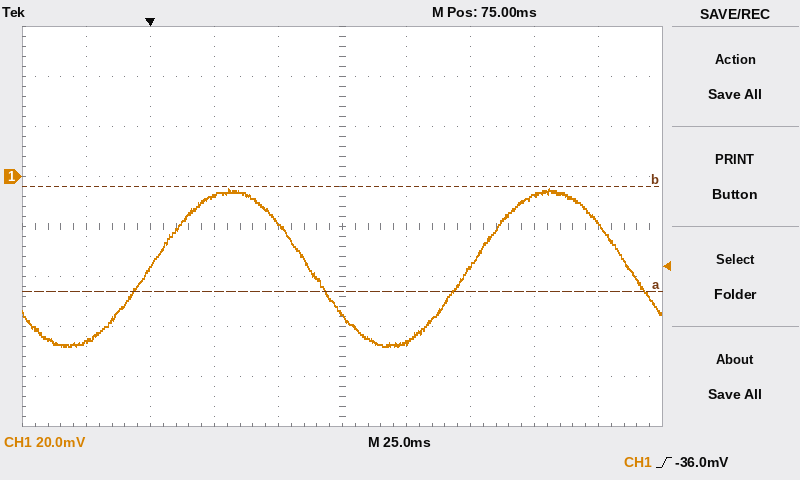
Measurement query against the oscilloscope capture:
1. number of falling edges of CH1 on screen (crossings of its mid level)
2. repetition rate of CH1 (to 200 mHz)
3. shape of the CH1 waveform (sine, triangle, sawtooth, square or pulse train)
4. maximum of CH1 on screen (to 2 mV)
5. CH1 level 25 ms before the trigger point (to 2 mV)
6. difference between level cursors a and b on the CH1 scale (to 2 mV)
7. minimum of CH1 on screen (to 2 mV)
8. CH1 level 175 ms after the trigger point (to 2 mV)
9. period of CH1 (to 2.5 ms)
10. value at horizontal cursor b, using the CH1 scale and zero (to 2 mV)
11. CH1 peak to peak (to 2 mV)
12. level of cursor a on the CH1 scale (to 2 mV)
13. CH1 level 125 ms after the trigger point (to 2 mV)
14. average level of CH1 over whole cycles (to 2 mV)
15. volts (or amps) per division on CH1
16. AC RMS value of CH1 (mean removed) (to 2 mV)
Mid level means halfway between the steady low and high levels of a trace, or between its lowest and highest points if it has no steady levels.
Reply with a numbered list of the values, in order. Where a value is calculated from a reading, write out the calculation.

1. 2
2. 1 / 125.0 ms ≈ 8.0 Hz
3. sine
4. -4 mV
5. -66 mV
6. 42 mV
7. -68 mV
8. -18 mV
9. 125.0 ms
10. -4 mV
11. -4 mV − (-68 mV) = 64 mV
12. -46 mV
13. -36 mV
14. (-4 mV + (-68 mV)) / 2 ≈ -36 mV
15. 20 mV
16. 64 mV / (2√2) ≈ 22.6 mV, so 22 mV to the nearest 2 mV
